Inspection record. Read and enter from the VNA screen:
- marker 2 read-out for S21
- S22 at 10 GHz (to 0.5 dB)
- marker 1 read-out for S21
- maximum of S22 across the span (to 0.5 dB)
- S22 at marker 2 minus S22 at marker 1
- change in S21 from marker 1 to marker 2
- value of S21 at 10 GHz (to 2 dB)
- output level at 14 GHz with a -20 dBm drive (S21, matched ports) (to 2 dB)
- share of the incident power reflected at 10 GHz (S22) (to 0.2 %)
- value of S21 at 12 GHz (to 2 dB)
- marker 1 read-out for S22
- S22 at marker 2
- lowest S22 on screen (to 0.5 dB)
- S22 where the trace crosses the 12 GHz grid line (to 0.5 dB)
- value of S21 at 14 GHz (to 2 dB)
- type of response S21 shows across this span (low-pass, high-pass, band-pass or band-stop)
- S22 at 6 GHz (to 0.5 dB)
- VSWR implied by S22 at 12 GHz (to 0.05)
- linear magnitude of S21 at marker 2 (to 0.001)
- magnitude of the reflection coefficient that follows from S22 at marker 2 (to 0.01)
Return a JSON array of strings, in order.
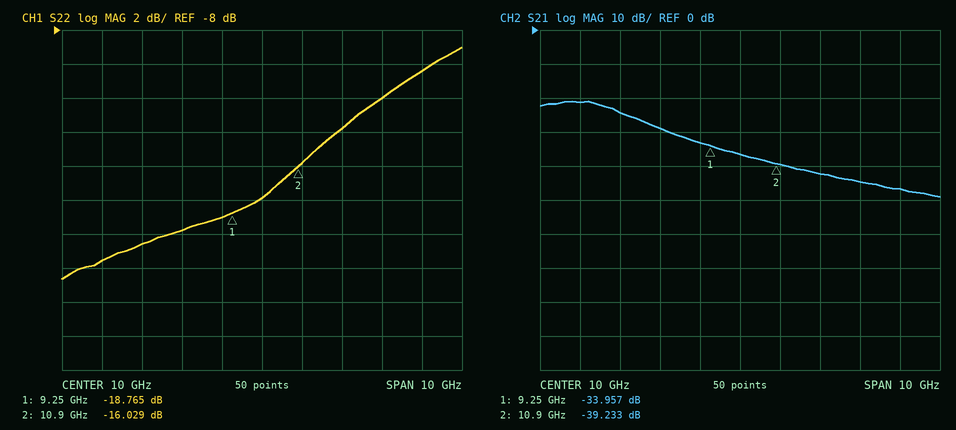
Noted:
["-39.233 dB", "-18.0 dB", "-33.957 dB", "-9.0 dB", "2.736 dB", "-5.276 dB", "-36 dB", "-66 dBm", "1.6 %", "-42 dB", "-18.765 dB", "-16.029 dB", "-22.5 dB", "-14.0 dB", "-46 dB", "low-pass", "-21.5 dB", "1.50", "0.011", "0.16"]
